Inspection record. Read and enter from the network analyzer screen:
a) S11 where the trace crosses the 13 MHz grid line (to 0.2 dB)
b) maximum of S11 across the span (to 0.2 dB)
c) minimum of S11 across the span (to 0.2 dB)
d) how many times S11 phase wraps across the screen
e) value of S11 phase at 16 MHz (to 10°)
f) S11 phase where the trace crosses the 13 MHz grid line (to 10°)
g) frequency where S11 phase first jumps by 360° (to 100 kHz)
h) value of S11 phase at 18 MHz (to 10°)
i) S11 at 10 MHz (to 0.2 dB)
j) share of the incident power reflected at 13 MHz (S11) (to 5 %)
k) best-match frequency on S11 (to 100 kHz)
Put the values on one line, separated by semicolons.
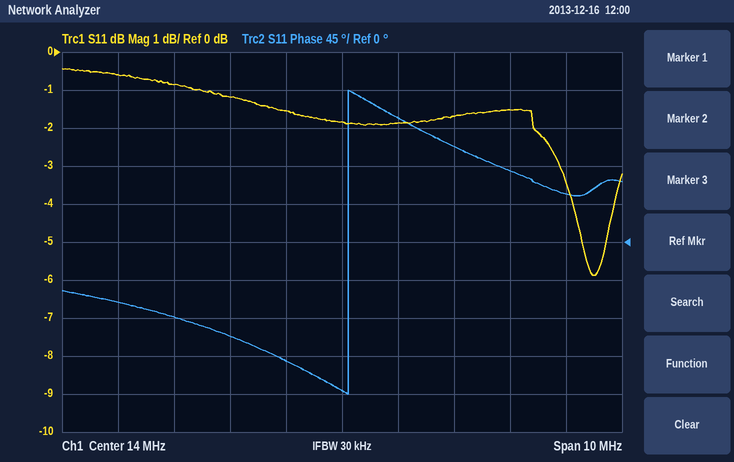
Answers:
-1.6 dB; -0.4 dB; -5.8 dB; 1; 110°; -140°; 14.1 MHz; 60°; -0.6 dB; 70 %; 18.5 MHz
